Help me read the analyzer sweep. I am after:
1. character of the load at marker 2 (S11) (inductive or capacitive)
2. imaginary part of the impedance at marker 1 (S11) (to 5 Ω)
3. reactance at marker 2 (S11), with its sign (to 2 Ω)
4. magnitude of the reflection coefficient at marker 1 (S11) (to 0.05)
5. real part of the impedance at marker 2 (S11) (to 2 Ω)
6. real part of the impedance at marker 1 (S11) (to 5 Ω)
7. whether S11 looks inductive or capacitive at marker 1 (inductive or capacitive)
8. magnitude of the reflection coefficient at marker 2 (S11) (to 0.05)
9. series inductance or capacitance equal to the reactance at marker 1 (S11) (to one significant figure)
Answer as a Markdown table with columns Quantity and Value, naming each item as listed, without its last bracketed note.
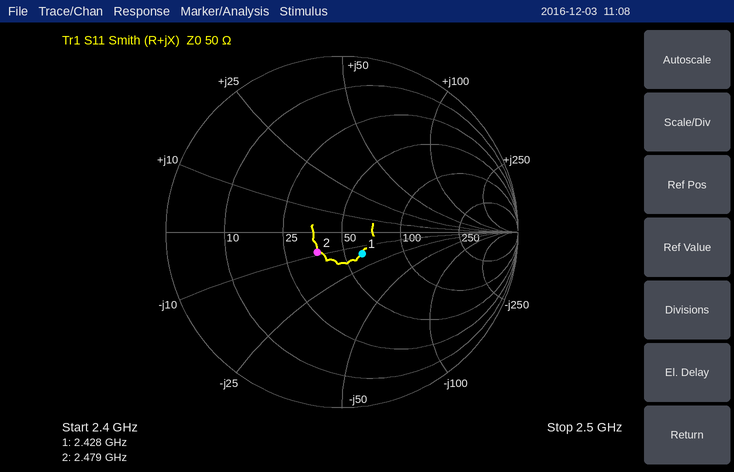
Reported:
| Quantity | Value |
|---|---|
| character of the load at marker 2 (S11) | capacitive |
| imaginary part of the impedance at marker 1 (S11) | -15 Ω |
| reactance at marker 2 (S11), with its sign | -8 Ω |
| magnitude of the reflection coefficient at marker 1 (S11) | 0.15 |
| real part of the impedance at marker 2 (S11) | 36 Ω |
| real part of the impedance at marker 1 (S11) | 60 Ω |
| whether S11 looks inductive or capacitive at marker 1 | capacitive |
| magnitude of the reflection coefficient at marker 2 (S11) | 0.20 |
| series inductance or capacitance equal to the reactance at marker 1 (S11) | 4 pF |
